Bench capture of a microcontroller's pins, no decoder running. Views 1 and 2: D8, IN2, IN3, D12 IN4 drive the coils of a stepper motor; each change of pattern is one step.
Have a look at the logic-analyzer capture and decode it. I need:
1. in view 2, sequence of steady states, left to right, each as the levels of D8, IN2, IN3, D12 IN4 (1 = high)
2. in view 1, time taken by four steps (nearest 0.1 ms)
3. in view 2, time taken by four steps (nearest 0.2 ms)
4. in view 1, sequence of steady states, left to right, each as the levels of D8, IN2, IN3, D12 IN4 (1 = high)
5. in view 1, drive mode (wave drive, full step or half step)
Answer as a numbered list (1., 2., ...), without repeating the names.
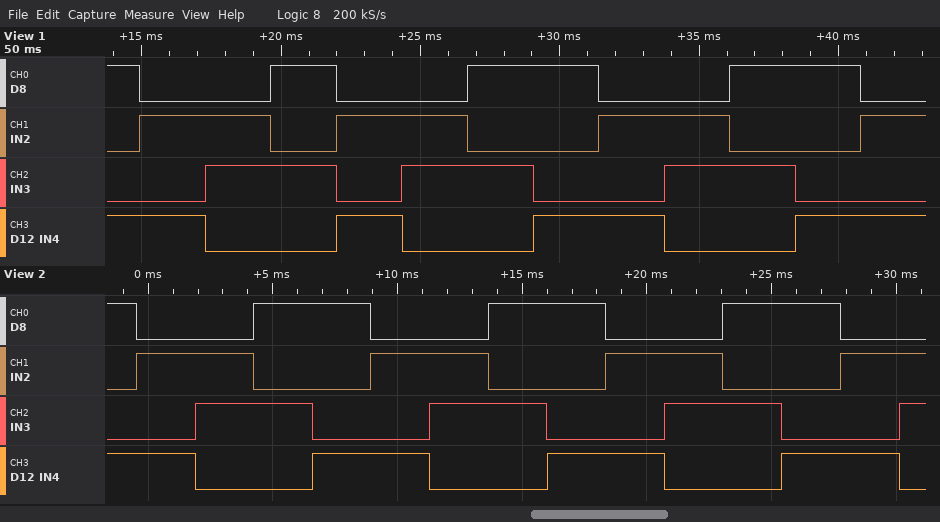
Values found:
1. 1001 0101 0110 1010 1001 0101 0110 1010 1001 0101 0110 1010 1001 0101 0110
2. 9.4 ms
3. 9.4 ms
4. 1001 0101 0110 1010 0101 0110 1010 1001 0101 0110 1010 1001 0101
5. full step
